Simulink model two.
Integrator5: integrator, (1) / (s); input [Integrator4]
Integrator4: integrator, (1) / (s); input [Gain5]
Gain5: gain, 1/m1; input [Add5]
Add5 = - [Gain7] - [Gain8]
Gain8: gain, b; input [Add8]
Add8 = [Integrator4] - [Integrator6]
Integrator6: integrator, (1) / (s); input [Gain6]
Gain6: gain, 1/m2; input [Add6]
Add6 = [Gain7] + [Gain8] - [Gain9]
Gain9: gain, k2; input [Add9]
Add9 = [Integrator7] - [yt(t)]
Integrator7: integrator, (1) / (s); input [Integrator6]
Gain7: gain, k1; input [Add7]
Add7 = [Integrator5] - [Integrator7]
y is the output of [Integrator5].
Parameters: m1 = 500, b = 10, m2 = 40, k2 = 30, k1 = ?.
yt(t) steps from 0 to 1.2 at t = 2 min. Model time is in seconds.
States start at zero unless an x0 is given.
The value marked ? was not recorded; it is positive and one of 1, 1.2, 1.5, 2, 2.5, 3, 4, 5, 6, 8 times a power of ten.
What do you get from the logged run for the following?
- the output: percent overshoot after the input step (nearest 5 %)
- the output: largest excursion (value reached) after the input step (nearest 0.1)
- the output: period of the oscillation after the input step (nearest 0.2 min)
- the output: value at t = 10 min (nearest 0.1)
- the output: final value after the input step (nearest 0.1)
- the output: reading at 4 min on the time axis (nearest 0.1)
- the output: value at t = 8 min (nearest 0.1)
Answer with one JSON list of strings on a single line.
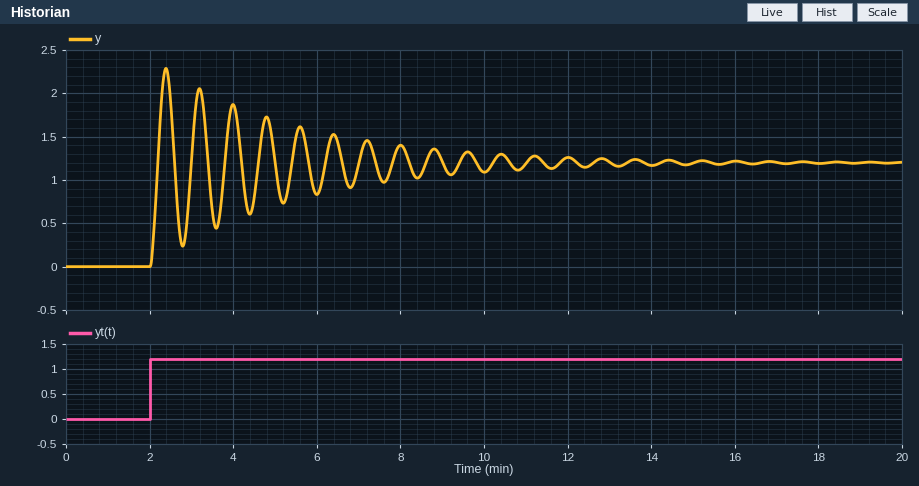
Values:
["90 %", "2.3", "0.8 min", "1.1", "1.2", "1.9", "1.4"]
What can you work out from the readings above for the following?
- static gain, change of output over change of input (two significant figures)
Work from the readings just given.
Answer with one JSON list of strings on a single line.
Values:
["1.0"]
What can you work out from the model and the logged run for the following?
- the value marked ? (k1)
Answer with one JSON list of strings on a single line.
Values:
["12"]
